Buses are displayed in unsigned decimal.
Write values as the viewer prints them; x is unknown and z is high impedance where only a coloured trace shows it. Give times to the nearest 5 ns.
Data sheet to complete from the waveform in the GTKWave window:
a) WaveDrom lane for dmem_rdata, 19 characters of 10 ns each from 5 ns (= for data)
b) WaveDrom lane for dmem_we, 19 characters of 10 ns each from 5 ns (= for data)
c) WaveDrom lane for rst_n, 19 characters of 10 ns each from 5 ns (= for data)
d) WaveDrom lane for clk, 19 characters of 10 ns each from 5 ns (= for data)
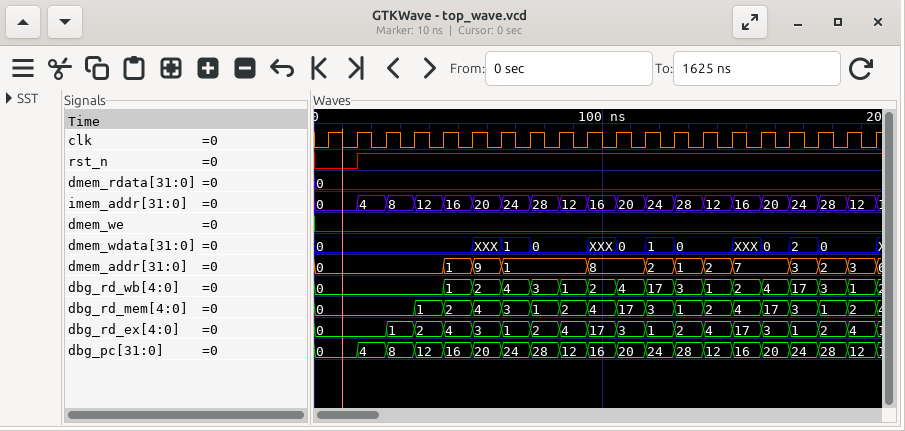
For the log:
{name: 'dmem_rdata', wave: '=..................', data: '0'}
{name: 'dmem_we', wave: '0..................'}
{name: 'rst_n', wave: '01.................'}
{name: 'clk', wave: 'p..................'}
